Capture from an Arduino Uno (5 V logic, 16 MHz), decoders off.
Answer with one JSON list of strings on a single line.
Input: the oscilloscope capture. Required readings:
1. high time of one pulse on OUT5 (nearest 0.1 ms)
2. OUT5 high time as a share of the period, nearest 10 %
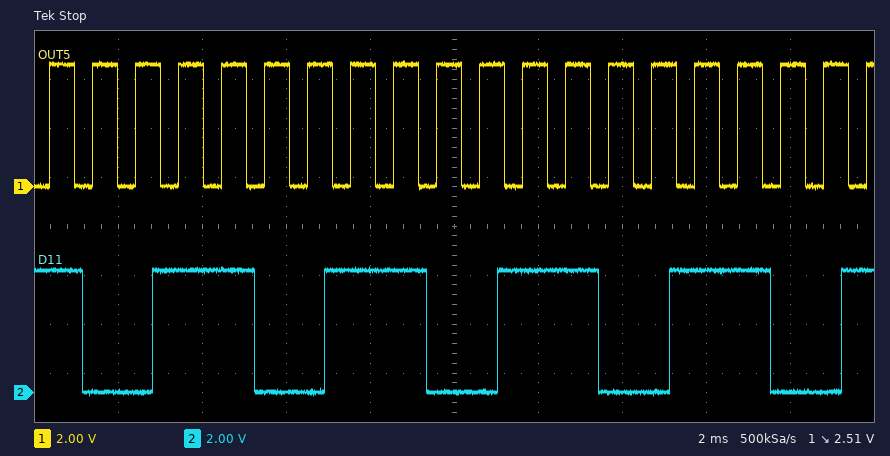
["0.6 ms", "60 %"]
